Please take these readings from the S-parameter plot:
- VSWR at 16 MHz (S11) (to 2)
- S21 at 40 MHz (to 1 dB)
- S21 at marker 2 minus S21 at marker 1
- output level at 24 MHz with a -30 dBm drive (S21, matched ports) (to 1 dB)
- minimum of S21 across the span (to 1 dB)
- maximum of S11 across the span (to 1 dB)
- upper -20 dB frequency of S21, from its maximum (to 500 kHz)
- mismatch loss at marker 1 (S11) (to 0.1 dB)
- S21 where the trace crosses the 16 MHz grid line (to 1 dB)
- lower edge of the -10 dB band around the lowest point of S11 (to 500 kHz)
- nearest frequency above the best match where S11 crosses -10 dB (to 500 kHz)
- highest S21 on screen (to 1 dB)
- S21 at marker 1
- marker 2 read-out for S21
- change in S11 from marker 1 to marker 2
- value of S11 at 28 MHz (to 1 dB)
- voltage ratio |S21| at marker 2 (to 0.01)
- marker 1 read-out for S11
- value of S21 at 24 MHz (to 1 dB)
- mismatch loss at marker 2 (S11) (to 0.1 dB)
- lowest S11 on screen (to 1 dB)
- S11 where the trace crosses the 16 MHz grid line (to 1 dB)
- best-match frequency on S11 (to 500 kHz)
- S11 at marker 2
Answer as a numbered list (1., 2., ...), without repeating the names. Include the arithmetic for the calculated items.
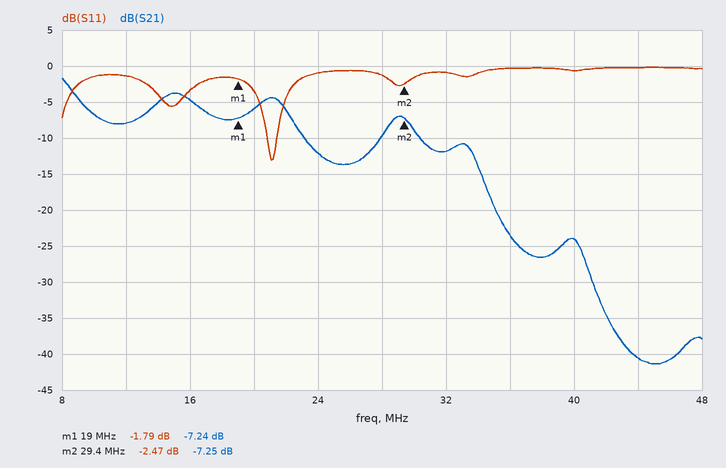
1. |Γ| = 10^(-3/20) = 0.7079; VSWR = (1 + 0.7079)/(1 − 0.7079) ≈ 6
2. -24 dB
3. -7.25 − (-7.24) = -0.01 dB
4. -30 dBm + (-12 dB) = -42 dBm
5. -41 dB
6. 0 dB
7. 35.5 MHz
8. −10 log10(1 − 10^(-1.79/10)) ≈ 4.7 dB
9. -5 dB
10. 21.0 MHz
11. 21.5 MHz
12. -2 dB
13. -7.24 dB
14. -7.25 dB
15. -2.47 − (-1.79) = -0.68 dB
16. -1 dB
17. 10^(-7.25/20) ≈ 0.43
18. -1.79 dB
19. -12 dB
20. −10 log10(1 − 10^(-2.47/10)) ≈ 3.6 dB
21. -13 dB
22. -3 dB
23. 21.0 MHz
24. -2.47 dB
